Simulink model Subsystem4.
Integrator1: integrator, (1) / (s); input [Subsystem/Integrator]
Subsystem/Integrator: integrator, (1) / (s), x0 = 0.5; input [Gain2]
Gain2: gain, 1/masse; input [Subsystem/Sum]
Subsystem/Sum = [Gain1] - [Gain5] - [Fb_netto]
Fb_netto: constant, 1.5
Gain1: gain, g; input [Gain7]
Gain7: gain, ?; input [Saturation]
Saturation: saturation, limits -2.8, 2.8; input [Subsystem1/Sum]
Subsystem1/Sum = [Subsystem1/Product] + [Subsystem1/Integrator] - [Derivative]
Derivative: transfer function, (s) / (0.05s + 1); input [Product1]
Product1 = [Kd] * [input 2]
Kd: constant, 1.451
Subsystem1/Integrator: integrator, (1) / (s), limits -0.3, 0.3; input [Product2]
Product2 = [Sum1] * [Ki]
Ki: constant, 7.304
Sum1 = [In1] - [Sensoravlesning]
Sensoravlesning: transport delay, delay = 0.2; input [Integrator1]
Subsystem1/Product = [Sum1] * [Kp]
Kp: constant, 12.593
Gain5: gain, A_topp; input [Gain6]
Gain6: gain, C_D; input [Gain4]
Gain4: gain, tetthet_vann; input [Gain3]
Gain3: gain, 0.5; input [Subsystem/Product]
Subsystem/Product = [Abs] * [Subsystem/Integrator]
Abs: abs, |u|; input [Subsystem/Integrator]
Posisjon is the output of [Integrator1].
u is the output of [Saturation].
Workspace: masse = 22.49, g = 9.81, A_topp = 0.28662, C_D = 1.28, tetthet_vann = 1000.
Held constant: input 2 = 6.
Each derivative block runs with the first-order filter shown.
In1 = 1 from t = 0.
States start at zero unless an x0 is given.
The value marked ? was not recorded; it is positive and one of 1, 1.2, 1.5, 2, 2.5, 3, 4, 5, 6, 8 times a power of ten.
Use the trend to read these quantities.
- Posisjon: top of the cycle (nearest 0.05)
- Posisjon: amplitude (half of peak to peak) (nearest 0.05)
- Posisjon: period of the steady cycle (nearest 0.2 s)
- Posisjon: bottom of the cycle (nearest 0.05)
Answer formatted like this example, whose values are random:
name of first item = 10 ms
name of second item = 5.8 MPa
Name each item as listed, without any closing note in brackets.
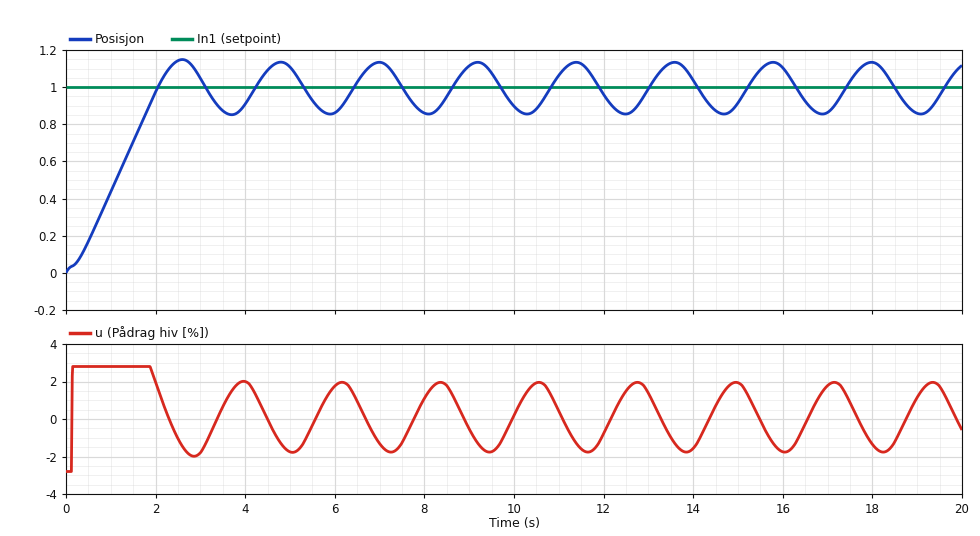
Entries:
Posisjon: top of the cycle = 1.15
Posisjon: amplitude (half of peak to peak) = 0.15
Posisjon: period of the steady cycle = 2.2 s
Posisjon: bottom of the cycle = 0.85
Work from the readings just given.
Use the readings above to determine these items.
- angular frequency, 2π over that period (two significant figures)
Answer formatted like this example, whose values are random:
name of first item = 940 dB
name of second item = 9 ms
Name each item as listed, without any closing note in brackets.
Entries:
angular frequency, 2π over that period = 2.9 rad/s
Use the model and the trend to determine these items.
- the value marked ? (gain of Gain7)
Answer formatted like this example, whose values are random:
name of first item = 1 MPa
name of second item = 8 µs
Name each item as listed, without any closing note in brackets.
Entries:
the value marked ? = 2
